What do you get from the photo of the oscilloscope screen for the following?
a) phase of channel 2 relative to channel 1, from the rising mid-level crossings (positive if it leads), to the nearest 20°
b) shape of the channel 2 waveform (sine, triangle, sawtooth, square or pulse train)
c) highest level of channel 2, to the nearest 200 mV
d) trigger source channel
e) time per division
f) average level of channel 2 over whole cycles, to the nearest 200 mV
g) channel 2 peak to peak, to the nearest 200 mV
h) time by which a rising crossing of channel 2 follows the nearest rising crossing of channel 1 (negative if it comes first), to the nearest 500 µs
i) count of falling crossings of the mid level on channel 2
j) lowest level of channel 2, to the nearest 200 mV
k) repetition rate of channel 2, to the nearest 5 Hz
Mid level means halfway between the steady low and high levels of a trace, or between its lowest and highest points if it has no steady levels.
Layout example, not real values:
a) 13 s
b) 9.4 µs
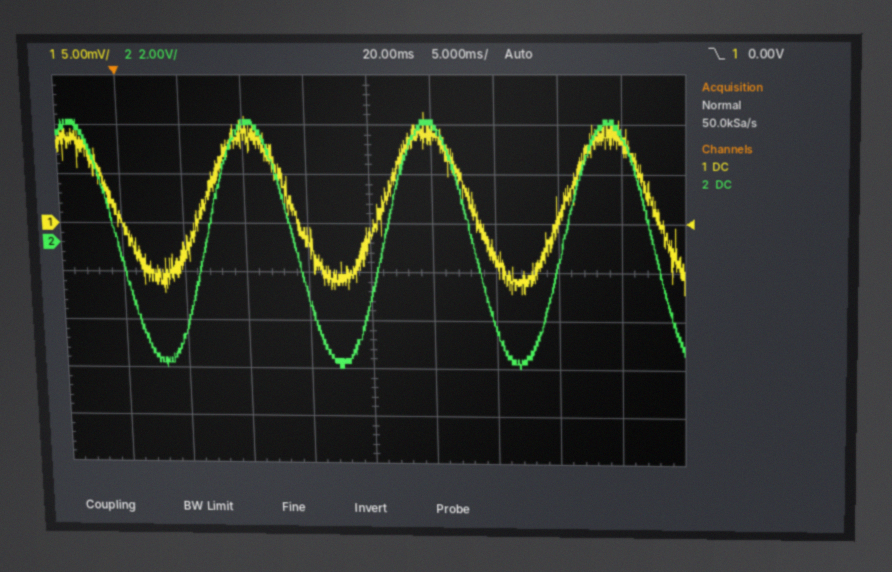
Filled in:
a) 0°
b) sine
c) 5.0 V
d) channel 1
e) 5 ms
f) 0.0 V
g) 10.2 V
h) 0.0 ms
i) 4
j) -5.2 V
k) 70 Hz
